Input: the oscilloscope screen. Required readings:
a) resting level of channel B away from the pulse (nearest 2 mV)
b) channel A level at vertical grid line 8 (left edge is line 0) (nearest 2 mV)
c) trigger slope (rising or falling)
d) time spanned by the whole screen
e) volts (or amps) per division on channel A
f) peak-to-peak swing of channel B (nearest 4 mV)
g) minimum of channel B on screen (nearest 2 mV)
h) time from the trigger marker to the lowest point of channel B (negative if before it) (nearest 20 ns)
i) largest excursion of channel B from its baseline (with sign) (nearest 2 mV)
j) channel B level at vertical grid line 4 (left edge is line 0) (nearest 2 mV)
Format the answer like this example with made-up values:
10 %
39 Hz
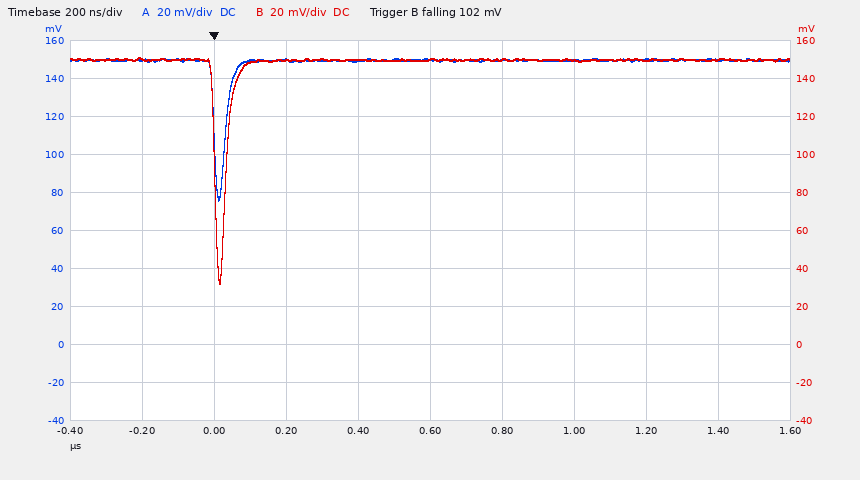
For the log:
150 mV
150 mV
falling
2 µs
20 mV
120 mV
32 mV
+20 ns
-118 mV
150 mV
